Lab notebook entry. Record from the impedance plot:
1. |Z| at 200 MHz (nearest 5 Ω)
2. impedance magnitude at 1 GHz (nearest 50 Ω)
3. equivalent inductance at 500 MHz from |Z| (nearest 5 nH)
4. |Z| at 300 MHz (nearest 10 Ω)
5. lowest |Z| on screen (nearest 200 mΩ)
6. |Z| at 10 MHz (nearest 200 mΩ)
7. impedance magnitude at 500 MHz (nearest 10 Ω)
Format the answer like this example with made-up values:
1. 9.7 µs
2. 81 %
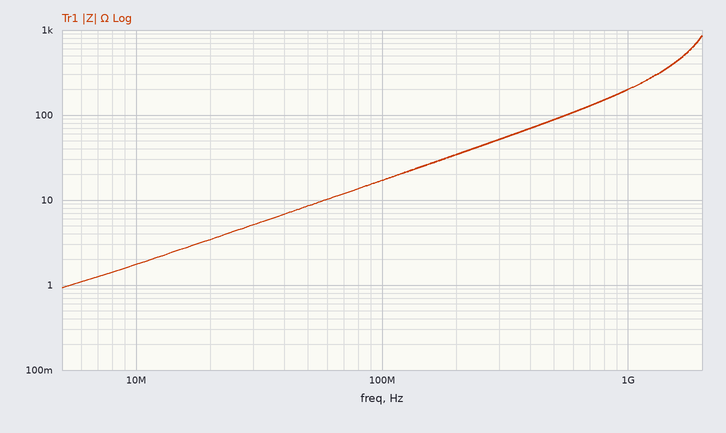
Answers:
1. 35 Ω
2. 200 Ω
3. 30 nH
4. 50 Ω
5. 1.0 Ω
6. 1.8 Ω
7. 90 Ω
